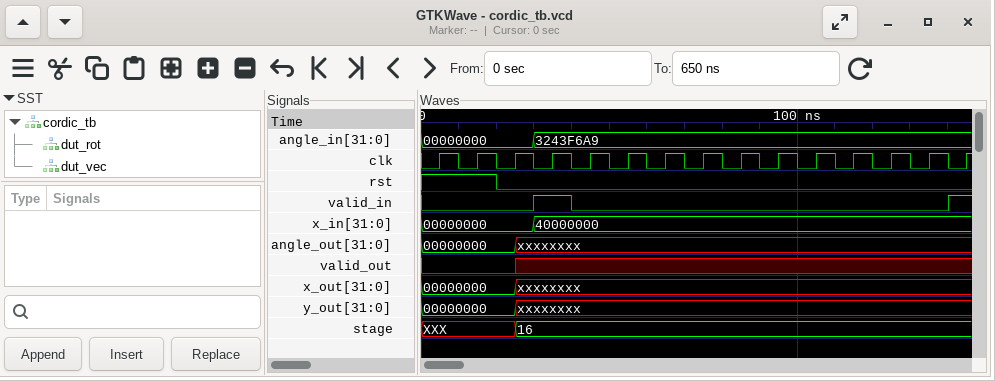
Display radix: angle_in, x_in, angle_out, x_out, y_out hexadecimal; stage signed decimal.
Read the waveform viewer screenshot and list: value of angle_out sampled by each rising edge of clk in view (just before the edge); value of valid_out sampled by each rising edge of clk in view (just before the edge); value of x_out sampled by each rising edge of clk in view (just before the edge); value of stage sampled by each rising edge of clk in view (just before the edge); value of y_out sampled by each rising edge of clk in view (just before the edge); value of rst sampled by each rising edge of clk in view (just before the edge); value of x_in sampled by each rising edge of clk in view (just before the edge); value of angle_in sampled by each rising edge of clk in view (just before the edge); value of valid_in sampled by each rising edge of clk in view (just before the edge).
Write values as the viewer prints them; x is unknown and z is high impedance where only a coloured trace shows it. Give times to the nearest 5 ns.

00000000, 00000000, 00000000, xxxxxxxx, xxxxxxxx, xxxxxxxx, xxxxxxxx, xxxxxxxx, xxxxxxxx, xxxxxxxx, xxxxxxxx, xxxxxxxx, xxxxxxxx, xxxxxxxx, xxxxxxxx
0 0 0 x x x x x x x x x x x x
00000000, 00000000, 00000000, xxxxxxxx, xxxxxxxx, xxxxxxxx, xxxxxxxx, xxxxxxxx, xxxxxxxx, xxxxxxxx, xxxxxxxx, xxxxxxxx, xxxxxxxx, xxxxxxxx, xxxxxxxx
XXX, XXX, XXX, 16, 16, 16, 16, 16, 16, 16, 16, 16, 16, 16, 16
00000000, 00000000, 00000000, xxxxxxxx, xxxxxxxx, xxxxxxxx, xxxxxxxx, xxxxxxxx, xxxxxxxx, xxxxxxxx, xxxxxxxx, xxxxxxxx, xxxxxxxx, xxxxxxxx, xxxxxxxx
1 1 0 0 0 0 0 0 0 0 0 0 0 0 0
00000000, 00000000, 00000000, 40000000, 40000000, 40000000, 40000000, 40000000, 40000000, 40000000, 40000000, 40000000, 40000000, 40000000, 40000000
00000000, 00000000, 00000000, 3243F6A9, 3243F6A9, 3243F6A9, 3243F6A9, 3243F6A9, 3243F6A9, 3243F6A9, 3243F6A9, 3243F6A9, 3243F6A9, 3243F6A9, 3243F6A9
0 0 0 1 0 0 0 0 0 0 0 0 0 0 1
